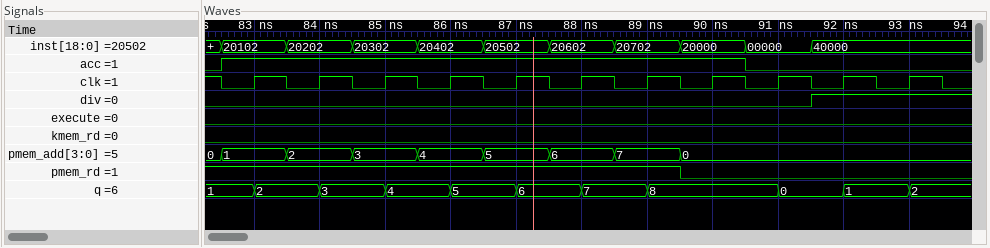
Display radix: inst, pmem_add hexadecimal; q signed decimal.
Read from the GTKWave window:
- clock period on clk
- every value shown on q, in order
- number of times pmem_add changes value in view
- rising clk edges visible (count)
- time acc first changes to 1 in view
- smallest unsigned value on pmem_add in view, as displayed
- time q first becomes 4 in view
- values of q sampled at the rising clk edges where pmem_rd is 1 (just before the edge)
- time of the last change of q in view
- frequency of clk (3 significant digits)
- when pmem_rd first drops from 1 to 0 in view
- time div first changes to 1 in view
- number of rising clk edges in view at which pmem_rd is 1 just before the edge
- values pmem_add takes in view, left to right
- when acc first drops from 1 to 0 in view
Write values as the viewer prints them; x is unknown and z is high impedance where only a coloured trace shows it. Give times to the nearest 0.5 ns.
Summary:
1 ns
1, 2, 3, 4, 5, 6, 7, 8, 0, 1, 2
8
11
82.5 ns
0
85 ns
1, 2, 3, 4, 5, 6, 7
93 ns
1.00 GHz
89.5 ns
91.5 ns
7
0, 1, 2, 3, 4, 5, 6, 7, 0
90.5 ns
